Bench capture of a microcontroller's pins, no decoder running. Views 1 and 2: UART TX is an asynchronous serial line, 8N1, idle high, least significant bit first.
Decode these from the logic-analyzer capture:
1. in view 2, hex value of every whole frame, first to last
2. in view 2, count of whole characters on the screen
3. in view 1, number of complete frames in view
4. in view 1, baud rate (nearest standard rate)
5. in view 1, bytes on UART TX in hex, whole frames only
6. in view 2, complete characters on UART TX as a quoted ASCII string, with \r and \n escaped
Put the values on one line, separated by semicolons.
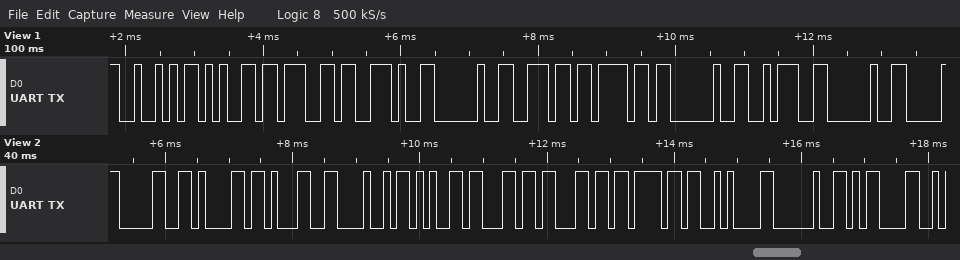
30 61 31 48 65 6C 6C 6F 0A 20 0D; 11; 10; 9600 baud; 52 65 67 2E 20 6E 6F 20 3A 20; "0a1Hello\n \r"
